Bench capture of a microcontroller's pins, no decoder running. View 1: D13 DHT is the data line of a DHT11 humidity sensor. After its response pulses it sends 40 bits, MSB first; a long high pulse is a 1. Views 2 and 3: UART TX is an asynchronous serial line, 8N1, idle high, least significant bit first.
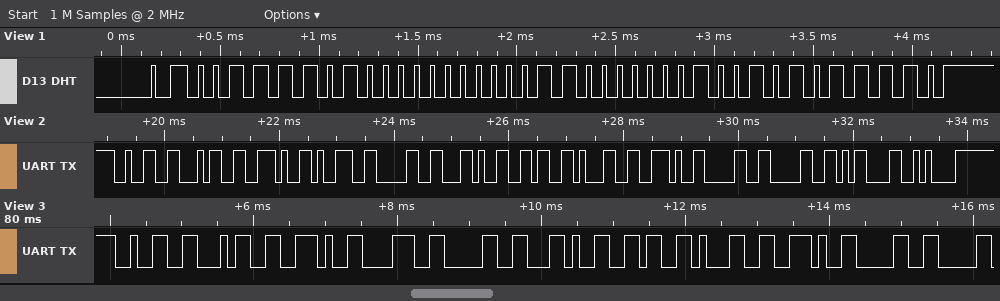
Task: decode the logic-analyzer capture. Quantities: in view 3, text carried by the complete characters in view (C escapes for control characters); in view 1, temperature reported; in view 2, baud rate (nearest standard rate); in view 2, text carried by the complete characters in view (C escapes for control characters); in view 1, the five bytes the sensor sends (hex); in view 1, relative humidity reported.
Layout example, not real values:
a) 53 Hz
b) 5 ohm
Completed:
a) "24.80,61.0"
b) 24.9 °C
c) 9600 baud
d) "24.90,61.00\r\n"
e) 3D 00 18 09 5E
f) 61 %
